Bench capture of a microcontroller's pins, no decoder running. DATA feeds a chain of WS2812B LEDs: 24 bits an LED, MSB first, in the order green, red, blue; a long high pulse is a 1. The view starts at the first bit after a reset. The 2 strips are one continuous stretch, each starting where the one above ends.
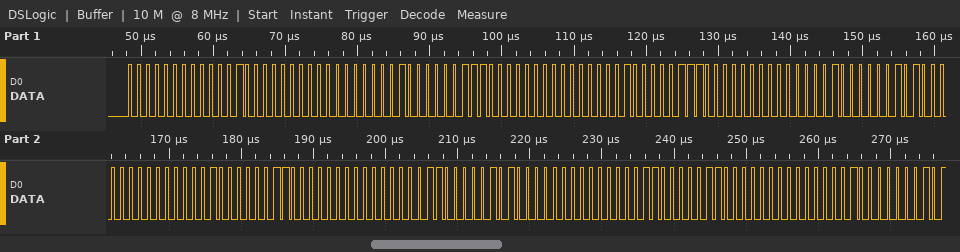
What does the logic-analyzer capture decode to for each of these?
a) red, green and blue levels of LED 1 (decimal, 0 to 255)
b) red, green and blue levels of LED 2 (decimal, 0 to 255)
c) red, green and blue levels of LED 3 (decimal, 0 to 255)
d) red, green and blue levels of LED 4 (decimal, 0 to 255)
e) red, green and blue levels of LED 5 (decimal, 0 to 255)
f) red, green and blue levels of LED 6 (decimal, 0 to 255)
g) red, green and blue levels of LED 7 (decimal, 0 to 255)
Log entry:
8, 0, 0
7, 2, 0
7, 1, 0
5, 2, 0
6, 2, 0
5, 3, 0
6, 3, 0
